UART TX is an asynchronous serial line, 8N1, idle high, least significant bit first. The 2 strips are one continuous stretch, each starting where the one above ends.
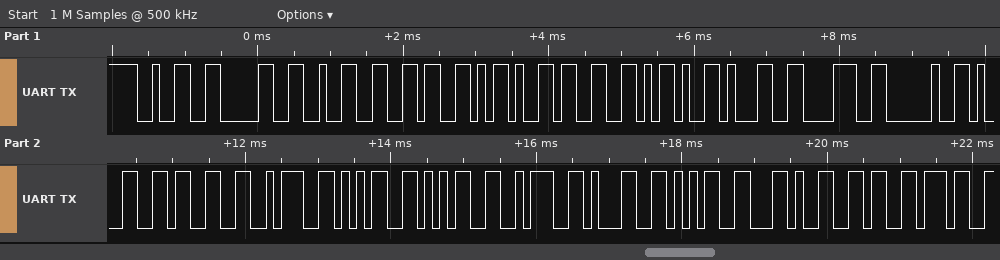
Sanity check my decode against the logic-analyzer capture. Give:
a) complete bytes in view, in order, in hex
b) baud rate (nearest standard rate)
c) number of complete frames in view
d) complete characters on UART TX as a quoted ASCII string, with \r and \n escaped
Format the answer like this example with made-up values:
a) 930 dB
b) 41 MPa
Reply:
a) 32 30 32 36 2D 33 2D 31 38 20 31 33 3A 35 35 3A 31 35 2C 36 37
b) 9600 baud
c) 21
d) "2026-3-18 13:55:15,67"
